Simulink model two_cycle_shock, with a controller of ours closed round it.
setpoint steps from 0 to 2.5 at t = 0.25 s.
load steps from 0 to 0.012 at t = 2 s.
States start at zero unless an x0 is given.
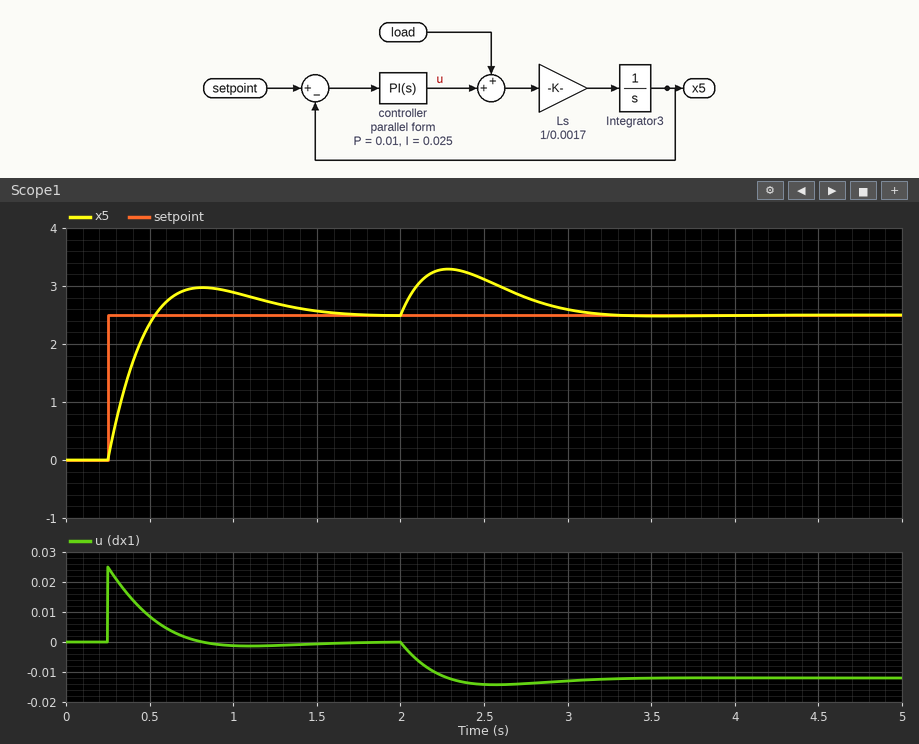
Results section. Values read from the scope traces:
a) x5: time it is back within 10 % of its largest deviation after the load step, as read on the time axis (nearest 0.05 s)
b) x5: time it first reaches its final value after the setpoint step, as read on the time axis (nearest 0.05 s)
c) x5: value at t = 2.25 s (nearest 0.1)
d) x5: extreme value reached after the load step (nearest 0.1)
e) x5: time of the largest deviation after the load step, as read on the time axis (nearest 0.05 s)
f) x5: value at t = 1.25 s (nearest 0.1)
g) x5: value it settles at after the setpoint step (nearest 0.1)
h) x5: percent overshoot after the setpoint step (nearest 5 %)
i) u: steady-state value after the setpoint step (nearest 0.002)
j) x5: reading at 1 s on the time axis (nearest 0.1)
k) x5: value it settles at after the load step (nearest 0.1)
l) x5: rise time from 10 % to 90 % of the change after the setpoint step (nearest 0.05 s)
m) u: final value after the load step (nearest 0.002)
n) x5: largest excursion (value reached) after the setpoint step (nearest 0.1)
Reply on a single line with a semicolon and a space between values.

3.05 s; 0.55 s; 3.3; 3.3; 2.30 s; 2.7; 2.5; 20 %; 0.000; 2.9; 2.5; 0.20 s; -0.012; 3.0
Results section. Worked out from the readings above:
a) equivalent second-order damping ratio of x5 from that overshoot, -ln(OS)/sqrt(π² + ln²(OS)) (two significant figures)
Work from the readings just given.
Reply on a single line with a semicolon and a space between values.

0.46
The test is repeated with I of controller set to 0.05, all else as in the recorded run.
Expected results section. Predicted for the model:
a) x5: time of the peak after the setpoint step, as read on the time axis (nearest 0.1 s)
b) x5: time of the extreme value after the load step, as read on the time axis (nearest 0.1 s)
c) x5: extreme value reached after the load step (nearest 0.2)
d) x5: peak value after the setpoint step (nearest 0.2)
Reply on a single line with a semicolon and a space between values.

0.7 s; 2.2 s; 3.2; 3.2
